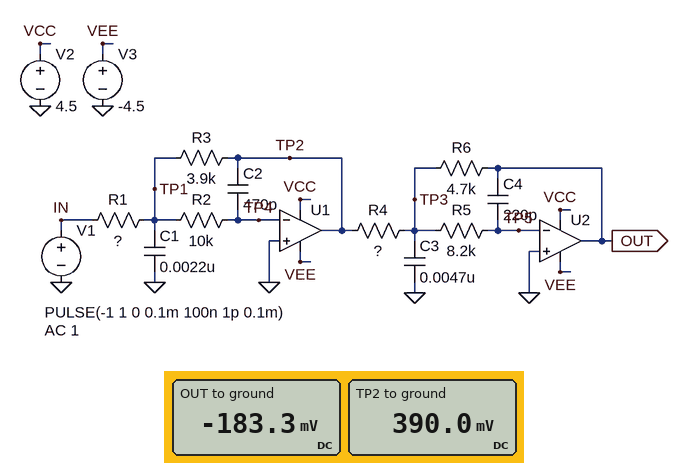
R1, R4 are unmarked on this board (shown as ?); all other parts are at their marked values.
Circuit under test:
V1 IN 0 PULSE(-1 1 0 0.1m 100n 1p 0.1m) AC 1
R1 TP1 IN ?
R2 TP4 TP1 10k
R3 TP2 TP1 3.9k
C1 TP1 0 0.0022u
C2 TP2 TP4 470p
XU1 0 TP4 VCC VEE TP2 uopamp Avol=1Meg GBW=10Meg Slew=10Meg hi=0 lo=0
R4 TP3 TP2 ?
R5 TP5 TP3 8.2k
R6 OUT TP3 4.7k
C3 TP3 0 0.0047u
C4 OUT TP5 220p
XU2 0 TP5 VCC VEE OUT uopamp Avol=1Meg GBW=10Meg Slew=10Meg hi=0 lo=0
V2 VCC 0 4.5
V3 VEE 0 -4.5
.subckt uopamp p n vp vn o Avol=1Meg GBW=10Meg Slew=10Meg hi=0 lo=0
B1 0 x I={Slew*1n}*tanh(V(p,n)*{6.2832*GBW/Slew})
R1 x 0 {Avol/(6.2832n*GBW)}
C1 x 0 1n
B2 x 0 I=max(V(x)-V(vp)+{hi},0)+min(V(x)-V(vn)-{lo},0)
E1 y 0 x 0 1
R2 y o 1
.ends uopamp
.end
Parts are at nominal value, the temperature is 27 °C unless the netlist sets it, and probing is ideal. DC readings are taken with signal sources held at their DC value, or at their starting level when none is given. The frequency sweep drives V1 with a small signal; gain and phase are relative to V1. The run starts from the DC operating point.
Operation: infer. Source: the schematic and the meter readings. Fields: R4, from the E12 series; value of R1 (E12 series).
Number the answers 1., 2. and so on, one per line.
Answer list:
1. 10 kΩ
2. 10 kΩ
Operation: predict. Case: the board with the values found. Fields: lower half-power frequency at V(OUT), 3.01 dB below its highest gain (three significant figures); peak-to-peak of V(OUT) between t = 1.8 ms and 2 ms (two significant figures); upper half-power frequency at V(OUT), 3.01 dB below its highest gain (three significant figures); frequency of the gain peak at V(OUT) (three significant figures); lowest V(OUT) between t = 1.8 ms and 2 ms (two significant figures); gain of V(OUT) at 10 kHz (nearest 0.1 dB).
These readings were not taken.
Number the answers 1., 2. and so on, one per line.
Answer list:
1. 7.22 kHz
2. 390 mV
3. 27.0 kHz
4. 20.8 kHz
5. -240 mV
6. -13.5 dB
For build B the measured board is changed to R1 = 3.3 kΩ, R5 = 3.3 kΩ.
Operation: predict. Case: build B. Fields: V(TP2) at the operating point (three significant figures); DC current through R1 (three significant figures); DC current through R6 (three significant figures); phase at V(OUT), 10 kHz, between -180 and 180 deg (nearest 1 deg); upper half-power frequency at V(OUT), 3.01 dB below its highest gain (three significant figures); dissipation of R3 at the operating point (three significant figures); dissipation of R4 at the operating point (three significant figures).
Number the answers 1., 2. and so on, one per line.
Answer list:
1. 1.18 V
2. 303 µA
3. 118 µA
4. -50 deg
5. 34.3 kHz
6. 358 µW
7. 140 µW
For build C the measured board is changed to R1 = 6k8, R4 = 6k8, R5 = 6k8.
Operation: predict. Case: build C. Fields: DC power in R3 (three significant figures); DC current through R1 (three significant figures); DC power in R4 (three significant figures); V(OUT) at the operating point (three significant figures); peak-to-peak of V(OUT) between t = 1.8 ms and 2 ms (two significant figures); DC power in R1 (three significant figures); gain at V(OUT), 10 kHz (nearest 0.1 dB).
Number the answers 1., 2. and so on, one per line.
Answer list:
1. 84.3 µW
2. 147 µA
3. 48.4 µW
4. -396 mV
5. 780 mV
6. 147 µW
7. -7.3 dB
